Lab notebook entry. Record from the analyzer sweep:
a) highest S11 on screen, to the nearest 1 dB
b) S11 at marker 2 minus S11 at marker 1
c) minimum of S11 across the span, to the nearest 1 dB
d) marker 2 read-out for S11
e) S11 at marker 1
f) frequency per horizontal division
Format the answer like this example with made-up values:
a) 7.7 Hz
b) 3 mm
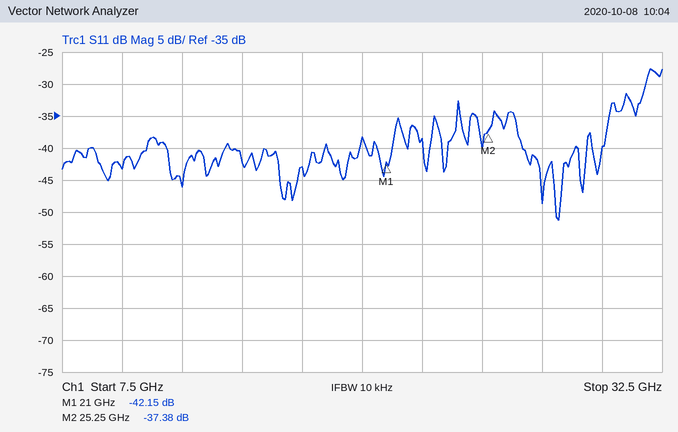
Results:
a) -28 dB
b) 4.77 dB
c) -51 dB
d) -37.38 dB
e) -42.15 dB
f) 2.5 GHz
